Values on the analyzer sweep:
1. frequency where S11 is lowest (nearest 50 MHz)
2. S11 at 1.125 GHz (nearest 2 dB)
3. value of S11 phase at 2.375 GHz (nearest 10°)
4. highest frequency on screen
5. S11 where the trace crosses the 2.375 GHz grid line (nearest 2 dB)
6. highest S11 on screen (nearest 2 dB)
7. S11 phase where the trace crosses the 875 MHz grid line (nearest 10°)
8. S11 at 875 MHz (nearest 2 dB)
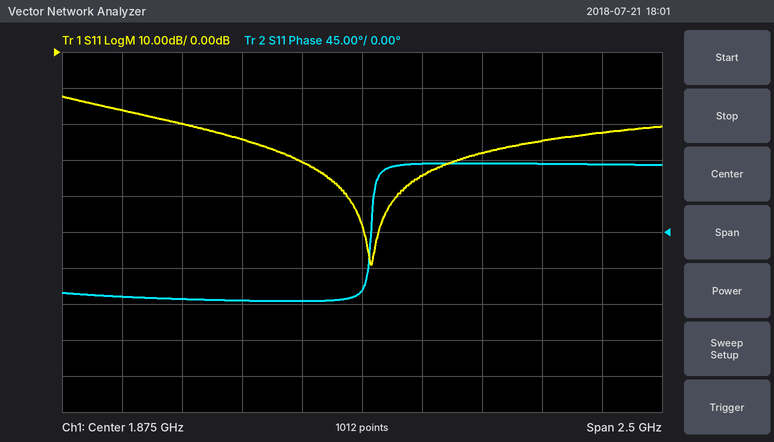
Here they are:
1.90 GHz
-20 dB
90°
3.125 GHz
-28 dB
-12 dB
-80°
-16 dB
